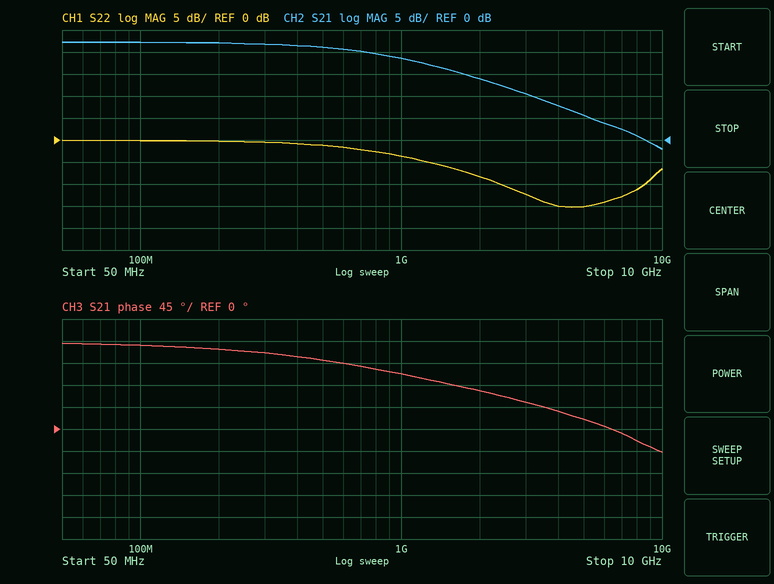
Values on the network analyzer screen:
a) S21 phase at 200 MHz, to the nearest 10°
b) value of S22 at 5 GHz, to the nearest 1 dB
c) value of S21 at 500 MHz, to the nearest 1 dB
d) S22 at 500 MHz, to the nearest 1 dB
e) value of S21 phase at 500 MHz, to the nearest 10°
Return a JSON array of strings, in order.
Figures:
["160°", "-15 dB", "21 dB", "-1 dB", "140°"]
